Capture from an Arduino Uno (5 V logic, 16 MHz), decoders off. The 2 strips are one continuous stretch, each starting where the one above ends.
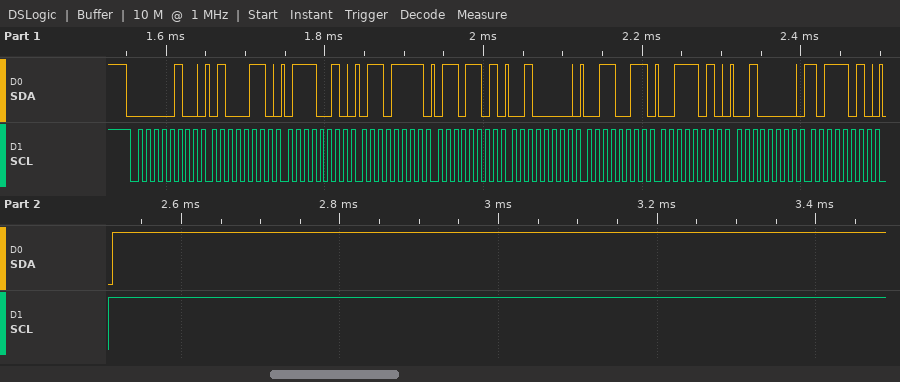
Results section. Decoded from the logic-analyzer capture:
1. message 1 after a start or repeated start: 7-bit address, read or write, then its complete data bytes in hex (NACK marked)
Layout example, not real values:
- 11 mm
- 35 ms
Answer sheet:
- 0x02 write: 46 72 6F 6D 20 33 3A 20 BA
